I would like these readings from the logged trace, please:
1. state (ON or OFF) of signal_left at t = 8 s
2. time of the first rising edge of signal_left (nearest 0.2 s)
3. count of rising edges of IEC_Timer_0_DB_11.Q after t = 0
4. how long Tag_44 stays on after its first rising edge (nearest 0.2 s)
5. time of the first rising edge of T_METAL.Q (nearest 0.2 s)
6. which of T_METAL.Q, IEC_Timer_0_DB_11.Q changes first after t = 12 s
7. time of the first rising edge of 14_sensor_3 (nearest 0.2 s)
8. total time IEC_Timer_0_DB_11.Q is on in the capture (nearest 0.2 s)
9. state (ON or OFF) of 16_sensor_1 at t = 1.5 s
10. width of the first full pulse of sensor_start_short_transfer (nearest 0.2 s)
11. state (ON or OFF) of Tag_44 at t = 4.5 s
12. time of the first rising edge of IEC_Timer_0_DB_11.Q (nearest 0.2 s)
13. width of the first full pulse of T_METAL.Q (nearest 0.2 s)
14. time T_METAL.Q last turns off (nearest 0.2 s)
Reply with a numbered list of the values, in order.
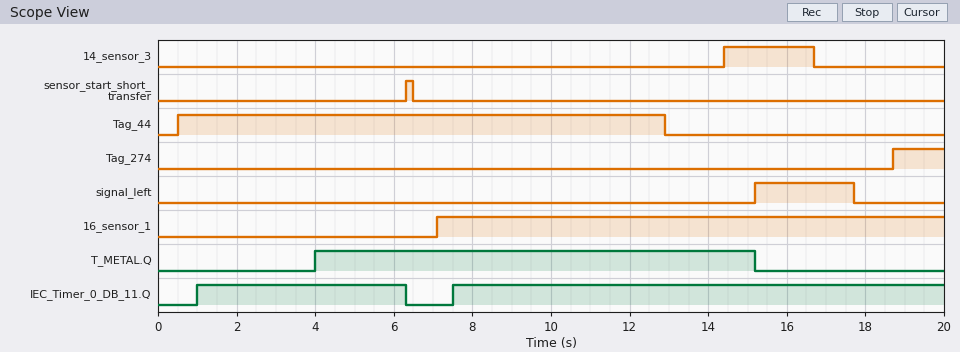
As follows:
1. OFF
2. 15.2 s
3. 2
4. 12.4 s
5. 4.0 s
6. T_METAL.Q
7. 14.4 s
8. 17.8 s
9. OFF
10. 0.2 s
11. ON
12. 1.0 s
13. 11.2 s
14. 15.2 s
